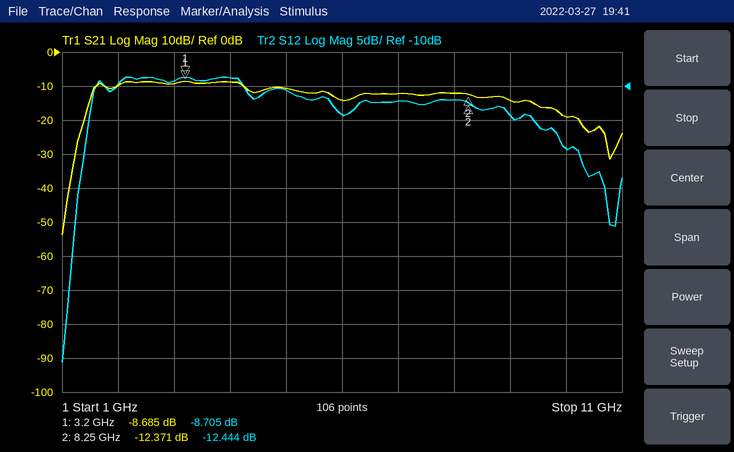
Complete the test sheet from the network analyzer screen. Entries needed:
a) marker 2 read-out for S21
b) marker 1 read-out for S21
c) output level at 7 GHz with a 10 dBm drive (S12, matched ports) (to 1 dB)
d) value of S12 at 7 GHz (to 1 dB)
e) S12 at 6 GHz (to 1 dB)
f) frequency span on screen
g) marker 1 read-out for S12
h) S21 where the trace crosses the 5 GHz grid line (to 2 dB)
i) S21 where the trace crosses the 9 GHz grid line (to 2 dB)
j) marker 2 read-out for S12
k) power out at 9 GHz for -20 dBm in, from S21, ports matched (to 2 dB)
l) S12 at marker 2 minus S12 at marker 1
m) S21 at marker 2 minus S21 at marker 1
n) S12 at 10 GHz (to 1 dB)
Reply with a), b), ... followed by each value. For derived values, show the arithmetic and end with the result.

a) -12.371 dB
b) -8.685 dB
c) 10 dBm + (-12 dB) = -2 dBm
d) -12 dB
e) -14 dB
f) 10 GHz
g) -8.705 dB
h) -10 dB
i) -14 dB
j) -12.444 dB
k) -20 dBm + (-14 dB) = -34 dBm
l) -12.444 − (-8.705) = -3.739 dB
m) -12.371 − (-8.685) = -3.686 dB
n) -19 dB
